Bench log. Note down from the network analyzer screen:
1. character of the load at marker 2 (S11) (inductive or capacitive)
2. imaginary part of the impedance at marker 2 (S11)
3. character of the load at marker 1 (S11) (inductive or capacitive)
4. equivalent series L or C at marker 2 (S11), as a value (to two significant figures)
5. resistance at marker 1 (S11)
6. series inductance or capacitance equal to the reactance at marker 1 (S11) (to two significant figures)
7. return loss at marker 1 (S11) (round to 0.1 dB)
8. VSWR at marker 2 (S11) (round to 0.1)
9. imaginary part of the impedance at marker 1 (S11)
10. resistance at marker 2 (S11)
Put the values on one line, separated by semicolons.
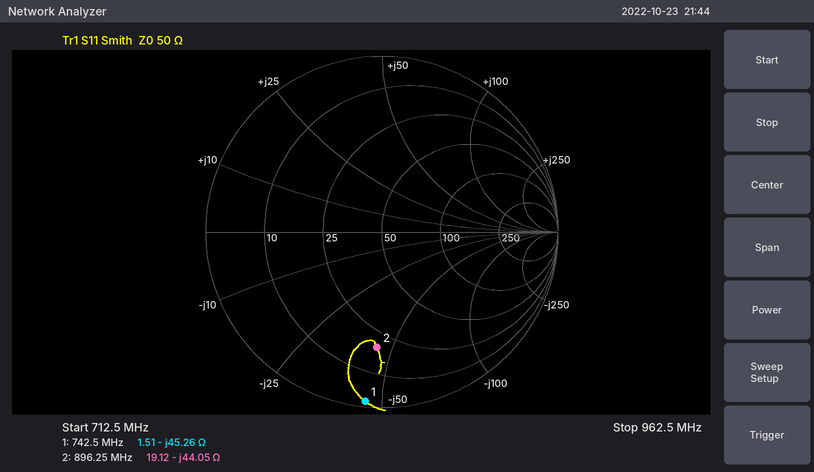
capacitive; -44.05 Ω; capacitive; 4.0 pF; 1.51 Ω; 4.7 pF; 0.3 dB; 4.8; -45.26 Ω; 19.12 Ω
